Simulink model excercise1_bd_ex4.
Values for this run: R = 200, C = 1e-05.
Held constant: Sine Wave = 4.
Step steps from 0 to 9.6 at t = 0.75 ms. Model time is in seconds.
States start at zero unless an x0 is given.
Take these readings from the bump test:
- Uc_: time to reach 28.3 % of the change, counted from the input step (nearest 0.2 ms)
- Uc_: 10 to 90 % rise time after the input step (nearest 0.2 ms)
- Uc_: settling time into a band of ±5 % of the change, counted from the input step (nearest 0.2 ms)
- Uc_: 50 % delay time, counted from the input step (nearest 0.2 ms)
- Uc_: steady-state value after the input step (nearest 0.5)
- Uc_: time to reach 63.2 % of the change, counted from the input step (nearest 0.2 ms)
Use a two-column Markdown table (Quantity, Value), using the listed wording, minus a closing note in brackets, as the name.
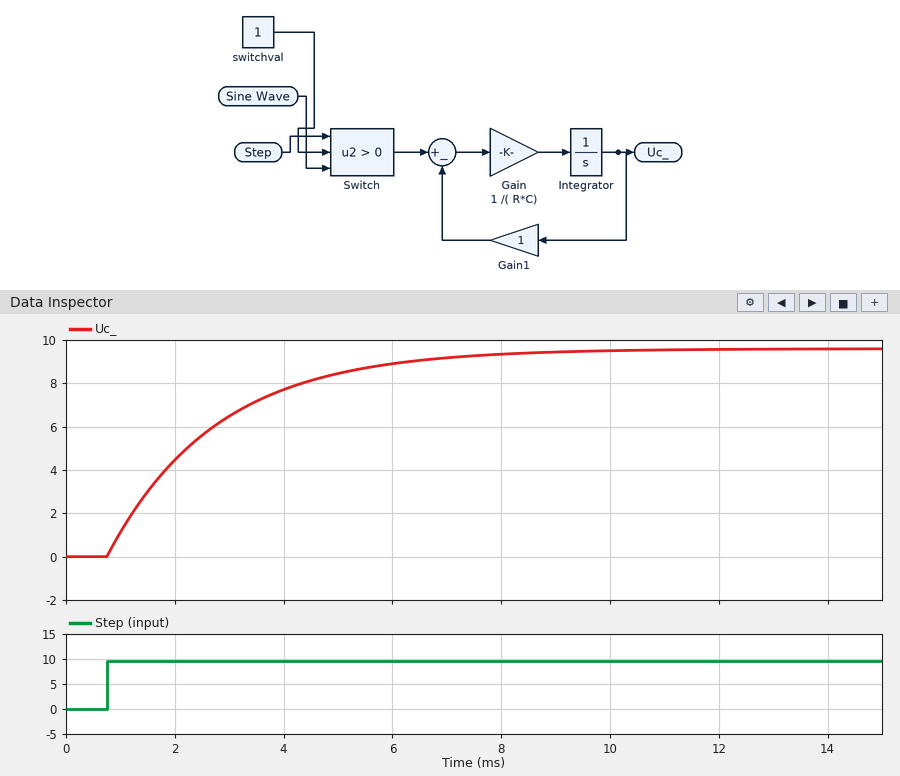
| Quantity | Value |
|---|---|
| Uc_: time to reach 28.3 % of the change, counted from the input step | 0.6 ms |
| Uc_: 10 to 90 % rise time after the input step | 4.4 ms |
| Uc_: settling time into a band of ±5 % of the change, counted from the input step | 6.0 ms |
| Uc_: 50 % delay time, counted from the input step | 1.4 ms |
| Uc_: steady-state value after the input step | 9.5 |
| Uc_: time to reach 63.2 % of the change, counted from the input step | 2.0 ms |
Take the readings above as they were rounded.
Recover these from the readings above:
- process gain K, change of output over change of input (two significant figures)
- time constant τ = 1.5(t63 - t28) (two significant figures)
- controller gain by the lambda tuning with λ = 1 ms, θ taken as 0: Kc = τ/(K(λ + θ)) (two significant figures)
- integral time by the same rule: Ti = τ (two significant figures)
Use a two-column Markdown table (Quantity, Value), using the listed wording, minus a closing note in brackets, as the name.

| Quantity | Value |
|---|---|
| process gain K, change of output over change of input | 0.99 |
| time constant τ = 1.5(t63 - t28) | 2.1 ms |
| controller gain by the lambda tuning with λ = 1 ms, θ taken as 0: Kc = τ/(K(λ + θ)) | 2.1 |
| integral time by the same rule: Ti = τ | 2.1 ms |
